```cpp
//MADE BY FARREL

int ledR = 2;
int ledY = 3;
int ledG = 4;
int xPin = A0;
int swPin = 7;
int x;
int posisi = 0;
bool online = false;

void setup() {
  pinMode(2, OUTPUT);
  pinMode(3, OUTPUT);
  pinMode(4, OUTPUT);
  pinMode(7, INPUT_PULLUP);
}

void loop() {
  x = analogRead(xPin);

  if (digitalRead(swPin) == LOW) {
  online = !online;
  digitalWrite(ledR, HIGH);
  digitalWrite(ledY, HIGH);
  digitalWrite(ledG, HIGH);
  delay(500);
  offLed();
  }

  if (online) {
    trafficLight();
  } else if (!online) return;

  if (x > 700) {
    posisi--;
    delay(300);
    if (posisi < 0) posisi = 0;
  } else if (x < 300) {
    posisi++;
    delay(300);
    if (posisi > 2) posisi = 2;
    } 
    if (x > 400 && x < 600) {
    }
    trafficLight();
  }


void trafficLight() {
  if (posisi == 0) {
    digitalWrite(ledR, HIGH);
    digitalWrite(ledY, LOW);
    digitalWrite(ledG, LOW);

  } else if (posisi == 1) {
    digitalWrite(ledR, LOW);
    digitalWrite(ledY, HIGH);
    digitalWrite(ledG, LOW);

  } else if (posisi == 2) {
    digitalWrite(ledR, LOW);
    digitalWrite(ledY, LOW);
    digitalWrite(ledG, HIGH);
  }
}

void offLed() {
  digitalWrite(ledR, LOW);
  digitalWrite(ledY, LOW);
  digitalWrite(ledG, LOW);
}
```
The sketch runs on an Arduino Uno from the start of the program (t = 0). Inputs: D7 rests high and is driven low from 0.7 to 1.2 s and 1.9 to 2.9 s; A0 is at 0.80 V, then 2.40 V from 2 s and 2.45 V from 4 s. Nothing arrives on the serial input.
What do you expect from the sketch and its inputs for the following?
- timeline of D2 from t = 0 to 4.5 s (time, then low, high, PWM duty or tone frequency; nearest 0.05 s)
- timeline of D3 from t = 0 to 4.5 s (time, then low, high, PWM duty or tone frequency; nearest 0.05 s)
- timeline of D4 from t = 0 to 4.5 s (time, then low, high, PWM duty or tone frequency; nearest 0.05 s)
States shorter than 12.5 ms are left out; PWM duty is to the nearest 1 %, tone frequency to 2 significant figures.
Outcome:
0 s low; 0.7 s high; 1.5 s low; 2.1 s high; 3.1 s low
0 s low; 0.7 s high; 1.2 s low; 1.5 s high; 1.8 s low; 2.1 s high; 3.1 s low
0 s low; 0.7 s high; 1.2 s low; 1.8 s high
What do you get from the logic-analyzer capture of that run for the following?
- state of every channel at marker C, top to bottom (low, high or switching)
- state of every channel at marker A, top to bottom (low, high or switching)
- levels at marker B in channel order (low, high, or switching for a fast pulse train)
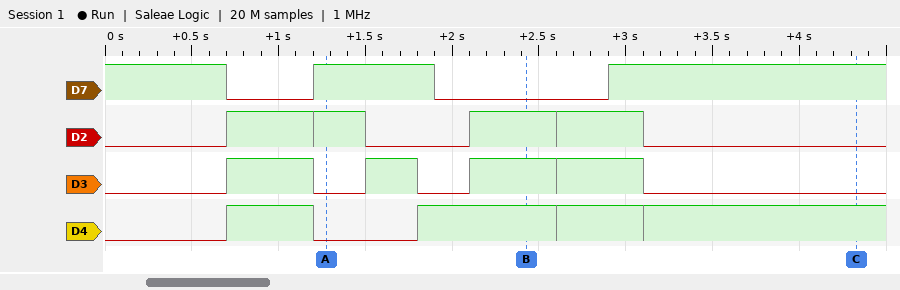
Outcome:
D7 high, D2 low, D3 low, D4 high
D7 high, D2 high, D3 low, D4 low
D7 low, D2 high, D3 high, D4 high
